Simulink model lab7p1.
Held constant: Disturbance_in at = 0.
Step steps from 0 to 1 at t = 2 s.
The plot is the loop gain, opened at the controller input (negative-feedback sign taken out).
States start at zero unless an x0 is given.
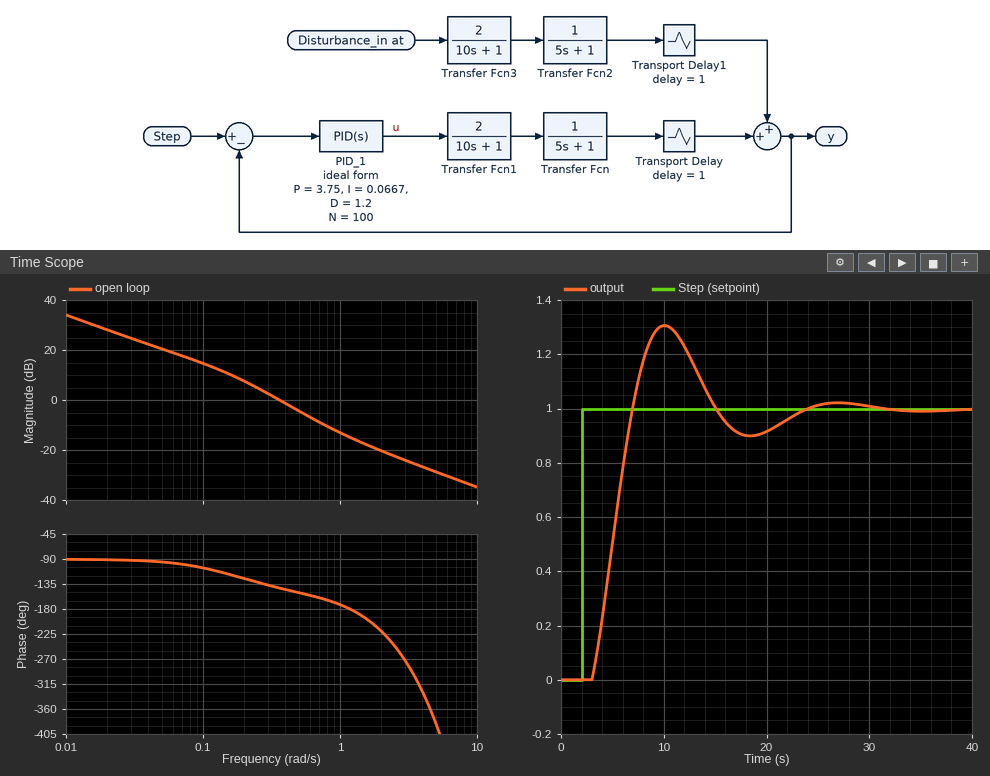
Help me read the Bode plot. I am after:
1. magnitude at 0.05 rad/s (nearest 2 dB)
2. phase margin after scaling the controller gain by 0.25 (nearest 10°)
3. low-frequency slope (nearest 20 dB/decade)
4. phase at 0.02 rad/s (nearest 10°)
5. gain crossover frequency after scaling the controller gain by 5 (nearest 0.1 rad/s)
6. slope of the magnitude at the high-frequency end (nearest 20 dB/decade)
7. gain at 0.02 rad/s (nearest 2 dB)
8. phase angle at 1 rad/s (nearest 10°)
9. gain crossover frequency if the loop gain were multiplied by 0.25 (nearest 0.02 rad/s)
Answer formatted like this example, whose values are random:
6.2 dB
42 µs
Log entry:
20 dB
70°
-20 dB/decade
-90°
1.1 rad/s
-20 dB/decade
28 dB
-170°
0.14 rad/s
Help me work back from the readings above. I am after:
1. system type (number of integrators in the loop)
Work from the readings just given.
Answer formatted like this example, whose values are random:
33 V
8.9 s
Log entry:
1
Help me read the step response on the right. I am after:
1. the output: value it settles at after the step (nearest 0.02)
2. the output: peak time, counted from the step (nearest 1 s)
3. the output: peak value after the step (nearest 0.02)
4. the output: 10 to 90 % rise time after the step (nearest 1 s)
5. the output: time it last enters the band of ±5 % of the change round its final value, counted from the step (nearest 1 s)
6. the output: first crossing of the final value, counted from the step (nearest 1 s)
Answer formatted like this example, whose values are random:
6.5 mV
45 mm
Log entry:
1.00
8 s
1.30
3 s
20 s
5 s
